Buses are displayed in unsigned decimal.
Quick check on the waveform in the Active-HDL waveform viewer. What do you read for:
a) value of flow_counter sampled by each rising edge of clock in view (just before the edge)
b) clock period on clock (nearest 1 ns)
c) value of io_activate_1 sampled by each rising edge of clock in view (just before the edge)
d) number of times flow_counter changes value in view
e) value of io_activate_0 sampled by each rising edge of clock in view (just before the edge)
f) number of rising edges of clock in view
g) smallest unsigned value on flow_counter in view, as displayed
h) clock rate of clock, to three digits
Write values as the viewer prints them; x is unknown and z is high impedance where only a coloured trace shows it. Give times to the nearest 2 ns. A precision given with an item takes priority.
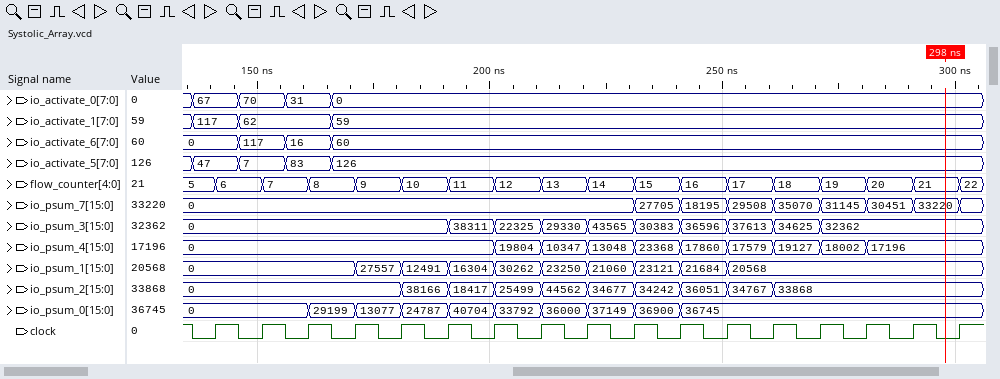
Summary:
5, 6, 7, 8, 9, 10, 11, 12, 13, 14, 15, 16, 17, 18, 19, 20, 21
10 ns
117, 62, 62, 59, 59, 59, 59, 59, 59, 59, 59, 59, 59, 59, 59, 59, 59
17
67, 70, 31, 0, 0, 0, 0, 0, 0, 0, 0, 0, 0, 0, 0, 0, 0
17
5
100 MHz
